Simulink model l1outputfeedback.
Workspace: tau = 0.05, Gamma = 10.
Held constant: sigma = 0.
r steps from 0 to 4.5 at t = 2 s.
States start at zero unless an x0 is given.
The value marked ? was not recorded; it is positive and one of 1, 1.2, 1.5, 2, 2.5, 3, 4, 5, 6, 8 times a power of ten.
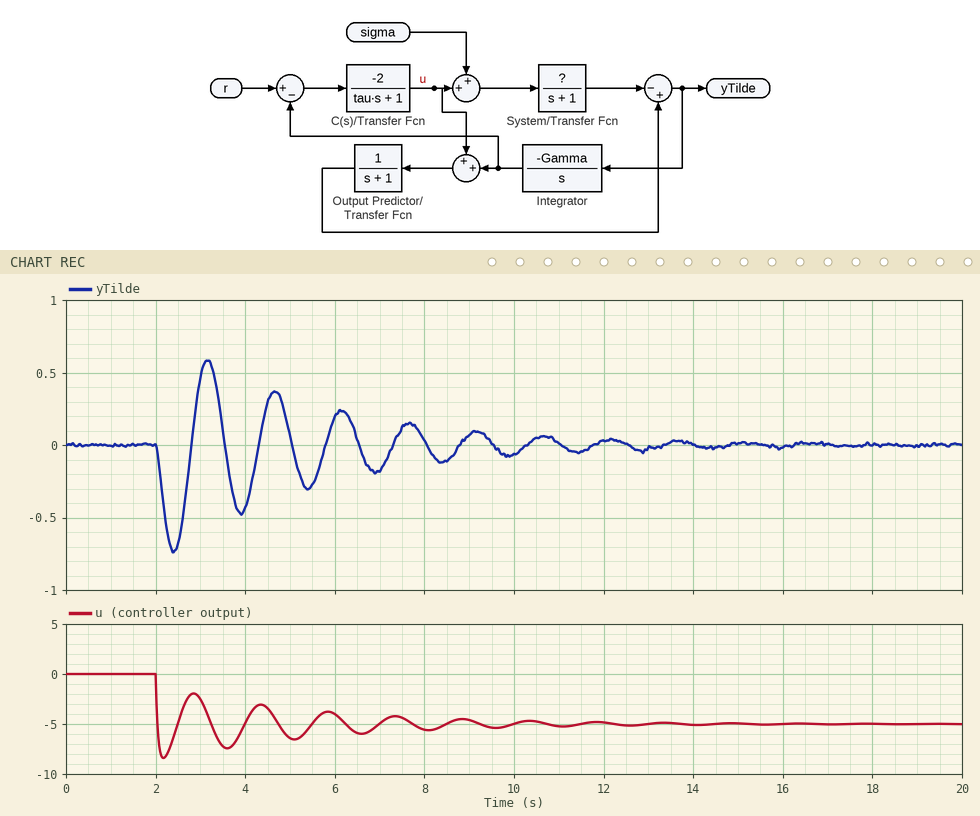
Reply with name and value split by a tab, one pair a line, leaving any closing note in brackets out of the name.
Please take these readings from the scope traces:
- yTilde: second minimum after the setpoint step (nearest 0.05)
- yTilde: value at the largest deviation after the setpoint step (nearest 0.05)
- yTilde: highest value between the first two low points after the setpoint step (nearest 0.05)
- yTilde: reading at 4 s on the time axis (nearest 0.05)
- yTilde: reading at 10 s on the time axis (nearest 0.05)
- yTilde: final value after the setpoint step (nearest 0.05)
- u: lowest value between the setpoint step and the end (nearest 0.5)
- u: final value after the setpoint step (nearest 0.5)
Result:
yTilde: second minimum after the setpoint step	-0.45
yTilde: value at the largest deviation after the setpoint step	-0.75
yTilde: highest value between the first two low points after the setpoint step	0.60
yTilde: reading at 4 s on the time axis	-0.45
yTilde: reading at 10 s on the time axis	-0.05
yTilde: final value after the setpoint step	0.00
u: lowest value between the setpoint step and the end	-8.5
u: final value after the setpoint step	-5.0
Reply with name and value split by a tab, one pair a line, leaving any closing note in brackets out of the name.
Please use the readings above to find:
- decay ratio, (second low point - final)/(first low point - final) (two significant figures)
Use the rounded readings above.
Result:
decay ratio, (second low point - final)/(first low point - final)	0.60
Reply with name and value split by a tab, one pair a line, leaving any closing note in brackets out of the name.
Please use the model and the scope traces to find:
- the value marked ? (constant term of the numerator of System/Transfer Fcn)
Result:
the value marked ?	0.6
